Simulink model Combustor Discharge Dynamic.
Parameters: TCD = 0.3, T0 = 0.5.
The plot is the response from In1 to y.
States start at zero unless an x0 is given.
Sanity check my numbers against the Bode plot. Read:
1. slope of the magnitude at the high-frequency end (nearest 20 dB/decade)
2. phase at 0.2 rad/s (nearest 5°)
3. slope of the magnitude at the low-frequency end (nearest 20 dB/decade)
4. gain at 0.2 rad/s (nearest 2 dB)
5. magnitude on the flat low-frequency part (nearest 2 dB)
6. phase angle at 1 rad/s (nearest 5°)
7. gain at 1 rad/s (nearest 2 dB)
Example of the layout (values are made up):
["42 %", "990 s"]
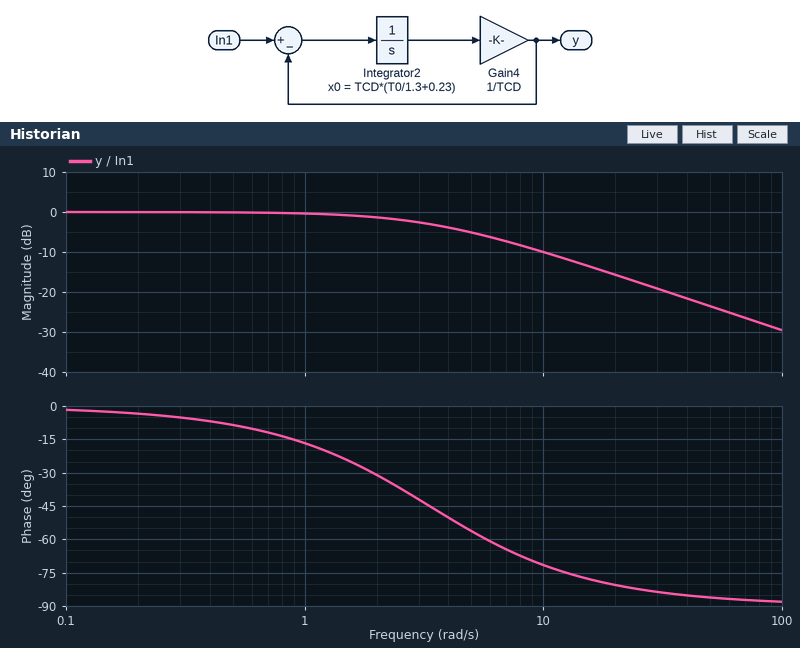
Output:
["-20 dB/decade", "-5°", "0 dB/decade", "0 dB", "0 dB", "-15°", "0 dB"]
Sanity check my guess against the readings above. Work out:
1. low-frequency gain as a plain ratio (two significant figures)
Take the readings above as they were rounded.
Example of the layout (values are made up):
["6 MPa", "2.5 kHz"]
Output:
["1.0"]
